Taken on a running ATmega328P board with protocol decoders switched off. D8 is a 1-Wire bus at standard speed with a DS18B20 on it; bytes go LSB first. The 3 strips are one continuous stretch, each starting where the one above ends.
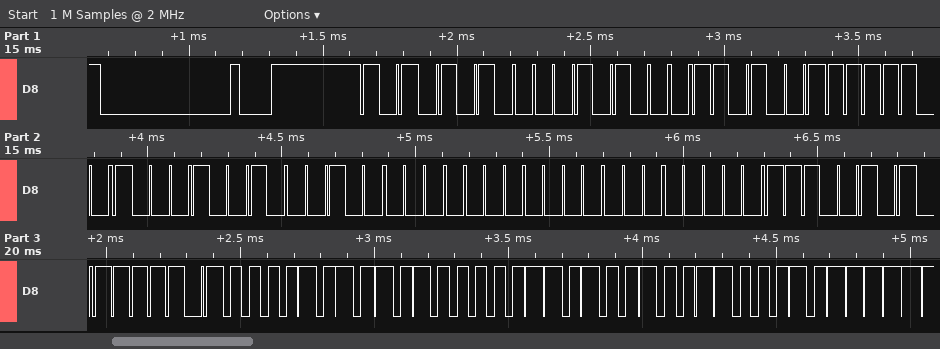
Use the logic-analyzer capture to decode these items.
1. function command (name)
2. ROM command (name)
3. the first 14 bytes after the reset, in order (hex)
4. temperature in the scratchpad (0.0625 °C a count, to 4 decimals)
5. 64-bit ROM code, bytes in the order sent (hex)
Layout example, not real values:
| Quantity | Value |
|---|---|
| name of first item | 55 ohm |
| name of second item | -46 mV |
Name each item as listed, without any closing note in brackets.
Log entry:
| Quantity | Value |
|---|---|
| function command | Read Scratchpad |
| ROM command | Match ROM |
| the first 14 bytes after the reset, in order | 55 28 96 9F 48 04 00 00 A7 BE 50 05 4B 46 |
| temperature in the scratchpad | 85.0000 °C |
| 64-bit ROM code, bytes in the order sent | 28 96 9F 48 04 00 00 A7 |
